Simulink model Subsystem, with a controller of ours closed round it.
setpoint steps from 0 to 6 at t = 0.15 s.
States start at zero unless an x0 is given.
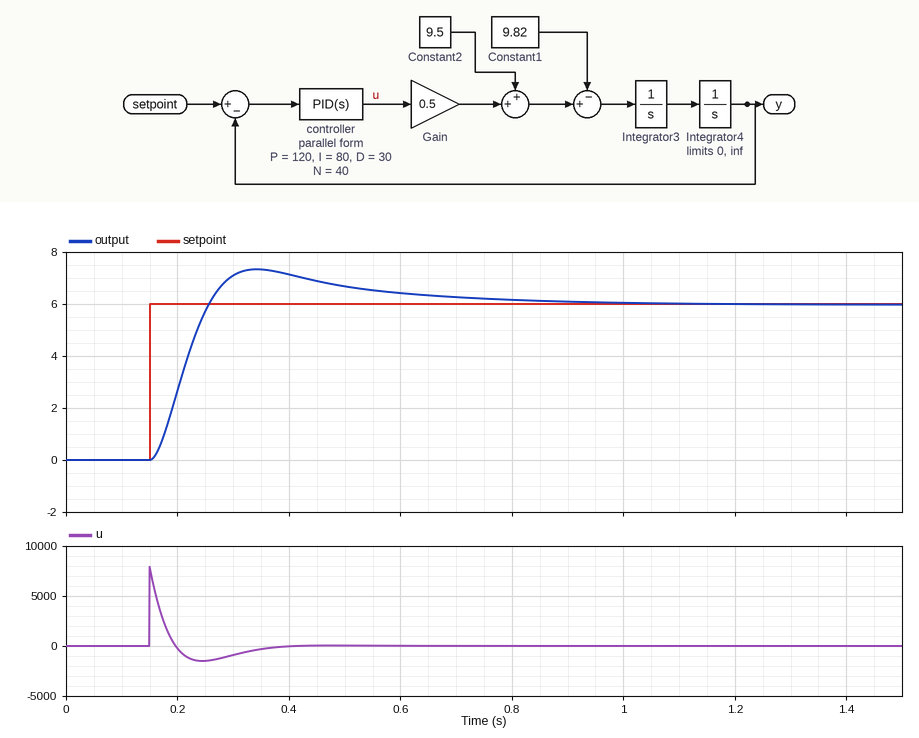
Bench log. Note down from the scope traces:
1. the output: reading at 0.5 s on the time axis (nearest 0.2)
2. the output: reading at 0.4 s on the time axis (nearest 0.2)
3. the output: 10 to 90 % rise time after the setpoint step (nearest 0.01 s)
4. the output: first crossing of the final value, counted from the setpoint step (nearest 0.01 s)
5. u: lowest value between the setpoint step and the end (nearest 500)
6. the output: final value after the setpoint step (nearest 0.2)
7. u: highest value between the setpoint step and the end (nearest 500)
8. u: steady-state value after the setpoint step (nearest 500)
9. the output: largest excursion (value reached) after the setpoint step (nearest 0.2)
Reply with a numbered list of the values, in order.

1. 6.6
2. 7.2
3. 0.07 s
4. 0.11 s
5. -1500
6. 6.0
7. 8000
8. 0
9. 7.4
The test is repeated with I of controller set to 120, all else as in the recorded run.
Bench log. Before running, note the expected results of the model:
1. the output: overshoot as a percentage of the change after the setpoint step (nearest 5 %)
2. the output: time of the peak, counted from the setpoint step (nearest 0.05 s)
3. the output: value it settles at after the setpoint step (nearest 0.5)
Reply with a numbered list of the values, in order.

1. 25 %
2. 0.20 s
3. 6.0
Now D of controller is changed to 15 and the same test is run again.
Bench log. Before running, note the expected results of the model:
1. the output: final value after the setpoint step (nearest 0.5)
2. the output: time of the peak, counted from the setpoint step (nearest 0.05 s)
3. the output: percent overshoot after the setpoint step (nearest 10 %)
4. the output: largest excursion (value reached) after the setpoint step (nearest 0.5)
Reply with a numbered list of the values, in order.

1. 6.0
2. 0.30 s
3. 40 %
4. 8.5
